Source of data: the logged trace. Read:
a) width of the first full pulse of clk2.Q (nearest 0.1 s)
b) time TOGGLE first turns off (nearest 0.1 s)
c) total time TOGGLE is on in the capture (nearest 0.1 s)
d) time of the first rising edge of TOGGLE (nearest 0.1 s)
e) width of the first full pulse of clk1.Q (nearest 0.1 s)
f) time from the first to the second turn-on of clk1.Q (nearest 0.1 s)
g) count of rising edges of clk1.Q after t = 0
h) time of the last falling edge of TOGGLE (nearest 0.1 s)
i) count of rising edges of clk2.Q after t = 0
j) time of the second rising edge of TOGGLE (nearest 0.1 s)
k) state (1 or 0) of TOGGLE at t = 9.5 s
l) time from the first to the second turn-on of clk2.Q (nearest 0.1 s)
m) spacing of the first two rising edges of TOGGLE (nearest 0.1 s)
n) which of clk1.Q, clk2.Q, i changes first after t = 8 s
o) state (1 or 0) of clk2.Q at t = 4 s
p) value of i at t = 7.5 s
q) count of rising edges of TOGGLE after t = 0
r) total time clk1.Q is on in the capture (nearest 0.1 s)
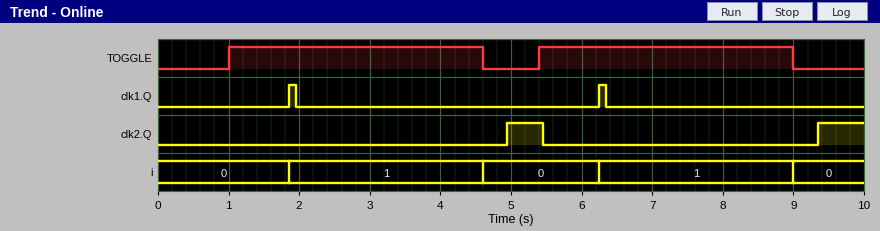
0.5 s
4.6 s
7.2 s
1.0 s
0.1 s
4.4 s
2
9.0 s
2
5.4 s
0
4.4 s
4.4 s
i
0
1
2
0.2 s
